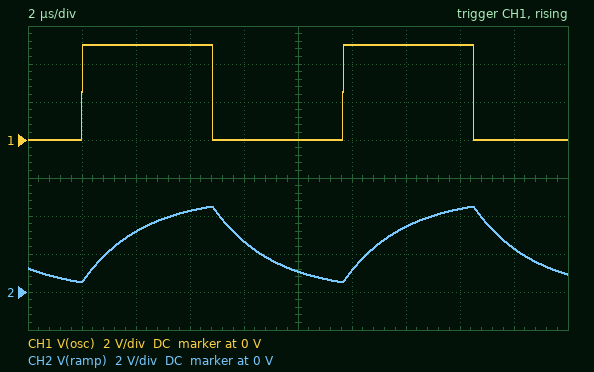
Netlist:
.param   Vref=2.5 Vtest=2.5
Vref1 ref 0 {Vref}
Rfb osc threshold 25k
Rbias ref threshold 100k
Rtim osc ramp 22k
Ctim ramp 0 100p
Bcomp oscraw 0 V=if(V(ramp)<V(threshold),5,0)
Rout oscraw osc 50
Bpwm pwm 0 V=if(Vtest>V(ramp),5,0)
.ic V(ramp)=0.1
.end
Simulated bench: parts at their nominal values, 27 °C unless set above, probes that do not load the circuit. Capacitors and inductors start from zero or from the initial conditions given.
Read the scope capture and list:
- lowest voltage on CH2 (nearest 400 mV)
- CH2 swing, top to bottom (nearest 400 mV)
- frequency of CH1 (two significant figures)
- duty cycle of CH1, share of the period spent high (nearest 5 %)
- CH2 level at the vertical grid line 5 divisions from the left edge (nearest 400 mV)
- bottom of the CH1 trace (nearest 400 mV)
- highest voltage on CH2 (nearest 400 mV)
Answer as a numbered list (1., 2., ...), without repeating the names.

1. 400 mV
2. 4.0 V
3. 100 kHz
4. 50 %
5. 1.2 V
6. 0 V
7. 4.4 V
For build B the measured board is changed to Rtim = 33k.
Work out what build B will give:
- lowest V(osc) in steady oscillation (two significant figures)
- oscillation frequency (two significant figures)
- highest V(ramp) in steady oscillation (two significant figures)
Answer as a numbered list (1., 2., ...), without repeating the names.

1. 1.8 mV
2. 69 kHz
3. 4.5 V
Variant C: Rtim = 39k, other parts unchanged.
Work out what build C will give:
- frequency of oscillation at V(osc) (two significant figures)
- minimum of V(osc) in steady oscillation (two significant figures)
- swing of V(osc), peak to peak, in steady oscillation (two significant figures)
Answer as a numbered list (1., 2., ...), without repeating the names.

1. 58 kHz
2. 1.6 mV
3. 5.0 V
